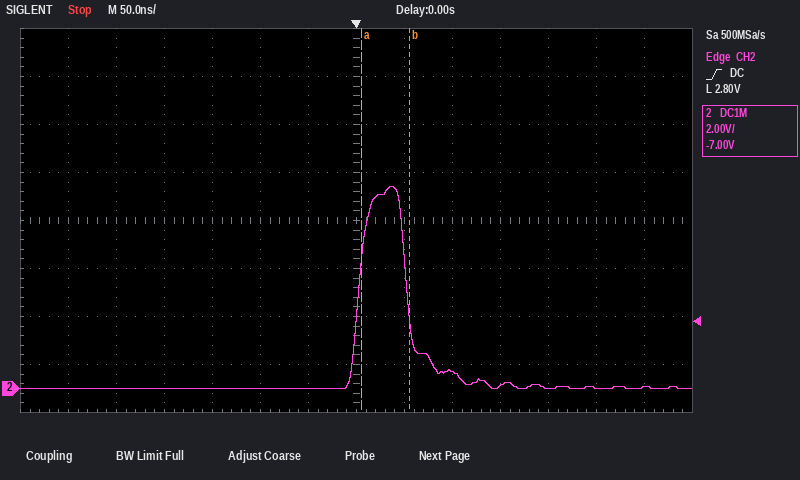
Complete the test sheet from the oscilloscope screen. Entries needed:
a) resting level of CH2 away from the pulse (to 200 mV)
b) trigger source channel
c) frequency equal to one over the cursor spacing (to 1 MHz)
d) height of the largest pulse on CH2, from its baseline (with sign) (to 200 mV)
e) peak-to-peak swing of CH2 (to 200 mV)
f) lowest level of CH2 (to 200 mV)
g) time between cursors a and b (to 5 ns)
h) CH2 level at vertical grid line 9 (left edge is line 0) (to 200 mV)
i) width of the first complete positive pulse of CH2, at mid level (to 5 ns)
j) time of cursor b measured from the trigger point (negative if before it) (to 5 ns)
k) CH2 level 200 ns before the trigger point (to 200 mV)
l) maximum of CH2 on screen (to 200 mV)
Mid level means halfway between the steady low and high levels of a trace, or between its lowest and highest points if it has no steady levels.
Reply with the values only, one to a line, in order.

0.0 V
CH2
20 MHz
+8.4 V
8.4 V
0.0 V
50 ns
800 mV
50 ns
+55 ns
0.0 V
8.4 V
